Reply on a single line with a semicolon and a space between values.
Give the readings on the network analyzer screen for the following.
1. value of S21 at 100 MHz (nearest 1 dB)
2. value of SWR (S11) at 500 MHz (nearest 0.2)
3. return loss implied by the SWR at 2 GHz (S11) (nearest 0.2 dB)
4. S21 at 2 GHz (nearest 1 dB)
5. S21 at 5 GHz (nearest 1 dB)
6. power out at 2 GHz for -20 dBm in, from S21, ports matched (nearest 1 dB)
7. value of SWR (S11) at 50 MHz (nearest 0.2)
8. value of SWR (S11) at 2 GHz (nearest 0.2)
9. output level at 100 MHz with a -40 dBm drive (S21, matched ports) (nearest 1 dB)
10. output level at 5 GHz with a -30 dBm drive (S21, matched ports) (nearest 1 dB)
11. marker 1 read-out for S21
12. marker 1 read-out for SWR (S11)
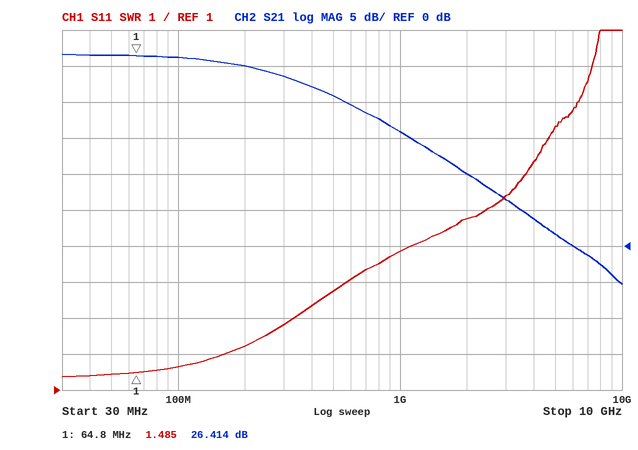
26 dB; 3.8; 3.0 dB; 10 dB; 2 dB; -10 dBm; 1.4; 5.8; -14 dBm; -28 dBm; 26.414 dB; 1.485
